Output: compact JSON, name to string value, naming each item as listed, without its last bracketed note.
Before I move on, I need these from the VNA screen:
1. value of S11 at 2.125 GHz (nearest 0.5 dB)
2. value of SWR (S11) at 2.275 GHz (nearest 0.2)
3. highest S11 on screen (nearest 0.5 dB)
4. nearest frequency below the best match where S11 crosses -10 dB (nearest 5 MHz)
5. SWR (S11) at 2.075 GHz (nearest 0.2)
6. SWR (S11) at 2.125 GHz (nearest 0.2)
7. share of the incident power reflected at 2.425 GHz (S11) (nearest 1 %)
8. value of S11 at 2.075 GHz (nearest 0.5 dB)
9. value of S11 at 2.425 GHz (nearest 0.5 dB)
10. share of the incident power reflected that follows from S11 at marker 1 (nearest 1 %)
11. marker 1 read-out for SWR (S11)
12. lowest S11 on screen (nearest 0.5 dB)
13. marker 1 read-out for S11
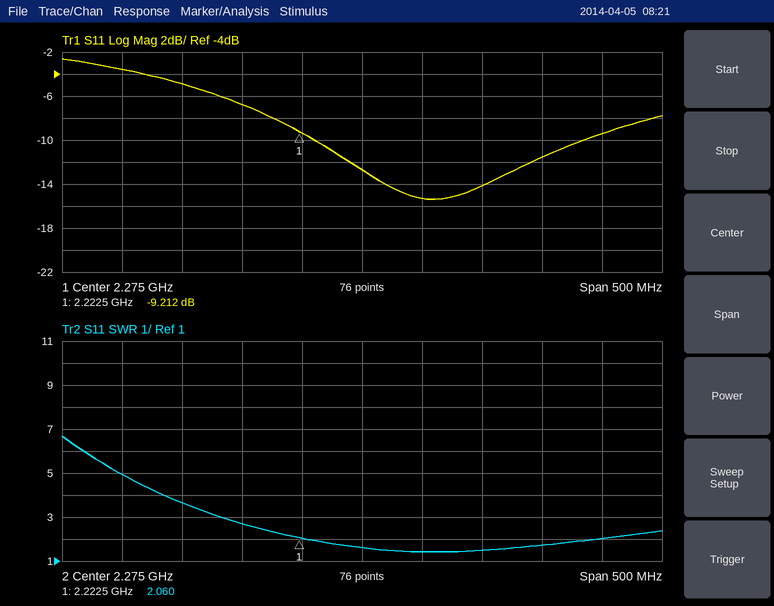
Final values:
{"value of S11 at 2.125 GHz": "-5.0 dB", "value of SWR (S11) at 2.275 GHz": "1.6", "highest S11 on screen": "-2.5 dB", "nearest frequency below the best match where S11 crosses -10 dB": "2.235 GHz", "SWR (S11) at 2.075 GHz": "5.0", "SWR (S11) at 2.125 GHz": "3.6", "share of the incident power reflected at 2.425 GHz (S11)": "7 %", "value of S11 at 2.075 GHz": "-3.5 dB", "value of S11 at 2.425 GHz": "-11.5 dB", "share of the incident power reflected that follows from S11 at marker 1": "12 %", "marker 1 read-out for SWR": "2.060", "lowest S11 on screen": "-15.5 dB", "marker 1 read-out for S11": "-9.212 dB"}
